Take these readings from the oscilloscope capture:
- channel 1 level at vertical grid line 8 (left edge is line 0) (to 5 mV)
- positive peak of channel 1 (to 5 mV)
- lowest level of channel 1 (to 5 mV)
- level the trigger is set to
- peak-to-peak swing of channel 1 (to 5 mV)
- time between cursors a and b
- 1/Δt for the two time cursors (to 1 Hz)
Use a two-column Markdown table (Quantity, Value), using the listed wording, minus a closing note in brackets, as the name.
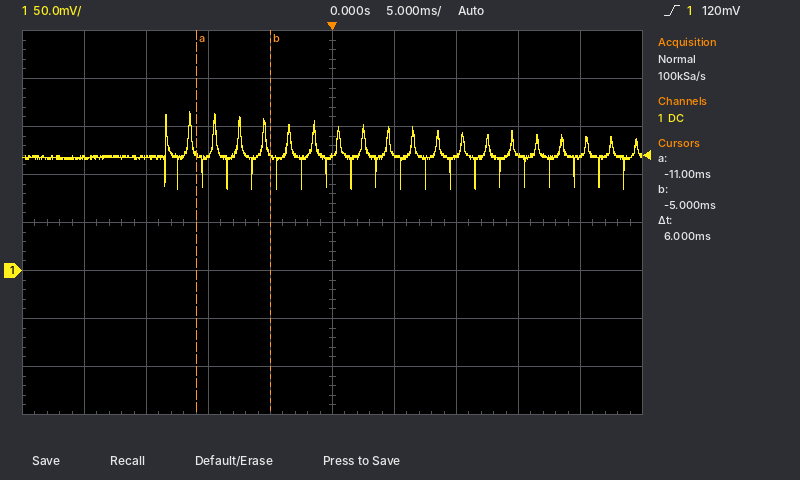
| Quantity | Value |
|---|---|
| channel 1 level at vertical grid line 8 (left edge is line 0) | 120 mV |
| positive peak of channel 1 | 165 mV |
| lowest level of channel 1 | 85 mV |
| level the trigger is set to | 120 mV |
| peak-to-peak swing of channel 1 | 80 mV |
| time between cursors a and b | 6 ms |
| 1/Δt for the two time cursors | 167 Hz |
